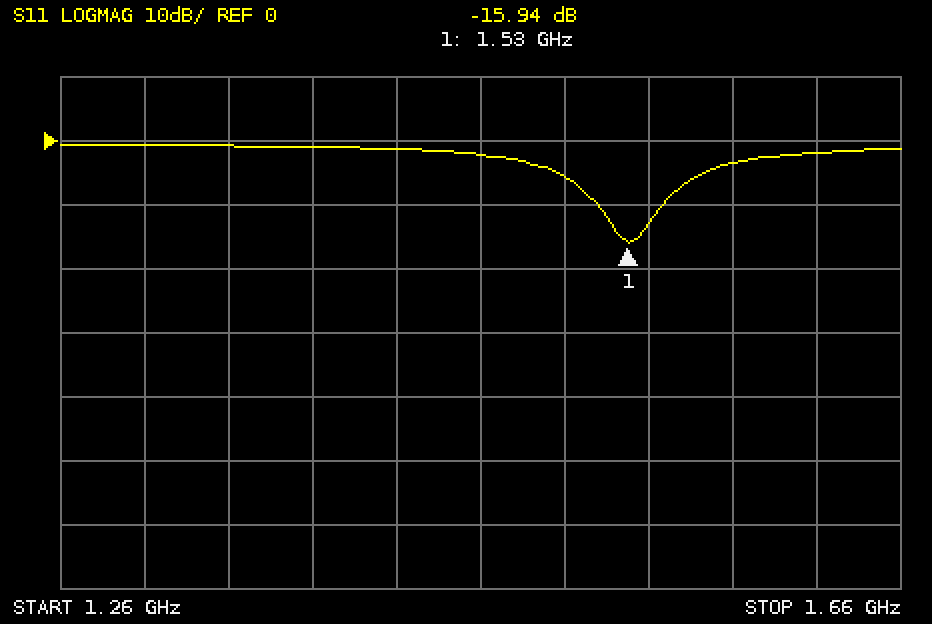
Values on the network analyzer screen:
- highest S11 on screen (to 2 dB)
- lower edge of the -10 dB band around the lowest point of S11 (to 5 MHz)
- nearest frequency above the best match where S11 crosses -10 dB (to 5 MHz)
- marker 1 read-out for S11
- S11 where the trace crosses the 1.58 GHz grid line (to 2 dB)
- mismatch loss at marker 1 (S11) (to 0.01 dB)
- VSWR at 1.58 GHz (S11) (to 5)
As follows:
0 dB
1.515 GHz
1.545 GHz
-15.94 dB
-4 dB
0.11 dB
5
